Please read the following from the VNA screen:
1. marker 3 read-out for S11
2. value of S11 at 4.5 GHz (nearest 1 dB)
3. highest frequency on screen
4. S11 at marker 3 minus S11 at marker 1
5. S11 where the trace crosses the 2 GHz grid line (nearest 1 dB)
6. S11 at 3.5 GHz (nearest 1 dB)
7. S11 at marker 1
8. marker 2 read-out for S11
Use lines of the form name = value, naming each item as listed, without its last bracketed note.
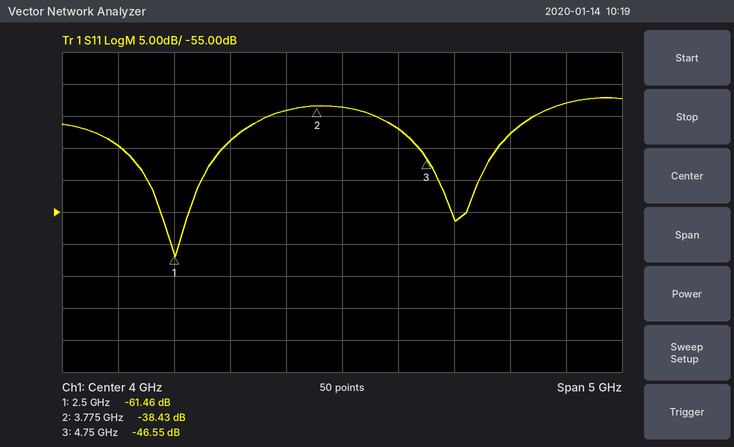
marker 3 read-out for S11 = -46.55 dB
value of S11 at 4.5 GHz = -42 dB
highest frequency on screen = 6.5 GHz
S11 at marker 3 minus S11 at marker 1 = 14.91 dB
S11 where the trace crosses the 2 GHz grid line = -45 dB
S11 at 3.5 GHz = -39 dB
S11 at marker 1 = -61.46 dB
marker 2 read-out for S11 = -38.43 dB
